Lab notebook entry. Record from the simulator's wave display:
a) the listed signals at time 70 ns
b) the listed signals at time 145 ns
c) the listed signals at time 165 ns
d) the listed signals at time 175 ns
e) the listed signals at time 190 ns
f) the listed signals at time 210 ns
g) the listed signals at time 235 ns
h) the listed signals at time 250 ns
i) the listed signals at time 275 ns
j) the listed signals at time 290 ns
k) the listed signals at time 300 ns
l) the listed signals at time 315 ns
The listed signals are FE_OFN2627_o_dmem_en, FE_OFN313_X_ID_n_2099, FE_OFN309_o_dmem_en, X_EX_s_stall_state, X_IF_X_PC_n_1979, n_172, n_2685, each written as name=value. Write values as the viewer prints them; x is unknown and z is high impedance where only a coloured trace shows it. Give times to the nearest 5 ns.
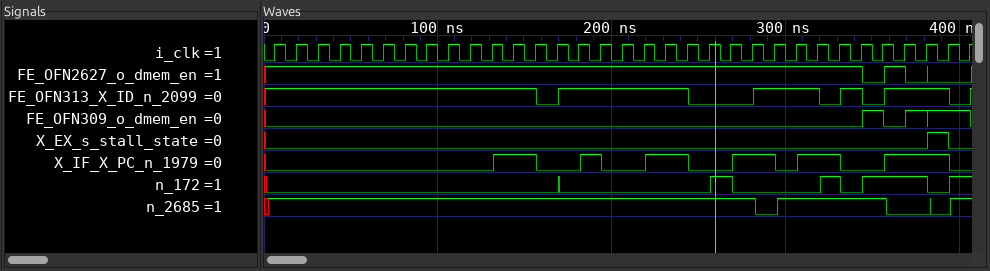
FE_OFN2627_o_dmem_en=1, FE_OFN313_X_ID_n_2099=1, FE_OFN309_o_dmem_en=0, X_EX_s_stall_state=0, X_IF_X_PC_n_1979=0, n_172=0, n_2685=1
FE_OFN2627_o_dmem_en=1, FE_OFN313_X_ID_n_2099=1, FE_OFN309_o_dmem_en=0, X_EX_s_stall_state=0, X_IF_X_PC_n_1979=1, n_172=0, n_2685=1
FE_OFN2627_o_dmem_en=1, FE_OFN313_X_ID_n_2099=0, FE_OFN309_o_dmem_en=0, X_EX_s_stall_state=0, X_IF_X_PC_n_1979=0, n_172=0, n_2685=1
FE_OFN2627_o_dmem_en=1, FE_OFN313_X_ID_n_2099=1, FE_OFN309_o_dmem_en=0, X_EX_s_stall_state=0, X_IF_X_PC_n_1979=0, n_172=0, n_2685=1
FE_OFN2627_o_dmem_en=1, FE_OFN313_X_ID_n_2099=1, FE_OFN309_o_dmem_en=0, X_EX_s_stall_state=0, X_IF_X_PC_n_1979=1, n_172=0, n_2685=1
FE_OFN2627_o_dmem_en=1, FE_OFN313_X_ID_n_2099=1, FE_OFN309_o_dmem_en=0, X_EX_s_stall_state=0, X_IF_X_PC_n_1979=0, n_172=0, n_2685=1
FE_OFN2627_o_dmem_en=1, FE_OFN313_X_ID_n_2099=1, FE_OFN309_o_dmem_en=0, X_EX_s_stall_state=0, X_IF_X_PC_n_1979=1, n_172=0, n_2685=1
FE_OFN2627_o_dmem_en=1, FE_OFN313_X_ID_n_2099=0, FE_OFN309_o_dmem_en=0, X_EX_s_stall_state=0, X_IF_X_PC_n_1979=0, n_172=0, n_2685=1
FE_OFN2627_o_dmem_en=1, FE_OFN313_X_ID_n_2099=0, FE_OFN309_o_dmem_en=0, X_EX_s_stall_state=0, X_IF_X_PC_n_1979=1, n_172=0, n_2685=1
FE_OFN2627_o_dmem_en=1, FE_OFN313_X_ID_n_2099=1, FE_OFN309_o_dmem_en=0, X_EX_s_stall_state=0, X_IF_X_PC_n_1979=1, n_172=0, n_2685=0
FE_OFN2627_o_dmem_en=1, FE_OFN313_X_ID_n_2099=1, FE_OFN309_o_dmem_en=0, X_EX_s_stall_state=0, X_IF_X_PC_n_1979=0, n_172=0, n_2685=1
FE_OFN2627_o_dmem_en=1, FE_OFN313_X_ID_n_2099=1, FE_OFN309_o_dmem_en=0, X_EX_s_stall_state=0, X_IF_X_PC_n_1979=1, n_172=0, n_2685=1
